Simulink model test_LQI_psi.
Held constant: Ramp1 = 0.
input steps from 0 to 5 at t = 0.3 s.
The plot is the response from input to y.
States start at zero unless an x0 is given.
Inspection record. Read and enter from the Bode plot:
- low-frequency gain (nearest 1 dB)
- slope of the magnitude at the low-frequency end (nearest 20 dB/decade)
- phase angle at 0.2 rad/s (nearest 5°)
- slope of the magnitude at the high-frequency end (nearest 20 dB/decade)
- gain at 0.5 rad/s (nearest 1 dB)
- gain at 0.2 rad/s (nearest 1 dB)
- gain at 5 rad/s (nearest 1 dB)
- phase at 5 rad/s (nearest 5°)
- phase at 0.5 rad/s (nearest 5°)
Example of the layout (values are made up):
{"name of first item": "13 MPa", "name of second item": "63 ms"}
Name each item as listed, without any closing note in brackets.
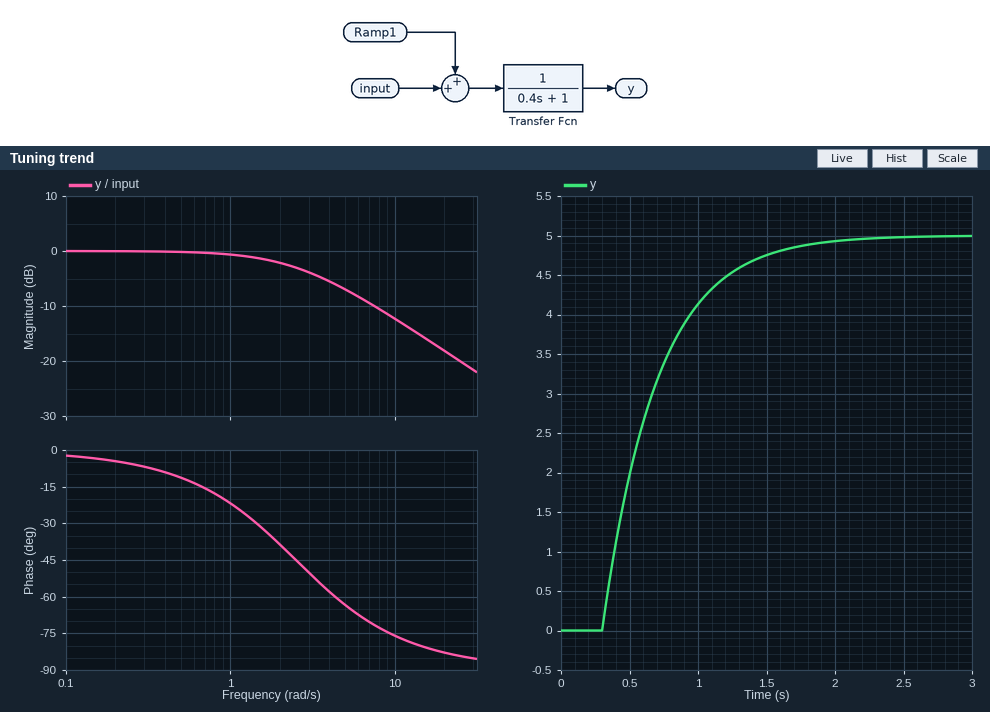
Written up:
{"low-frequency gain": "0 dB", "slope of the magnitude at the low-frequency end": "0 dB/decade", "phase angle at 0.2 rad/s": "-5°", "slope of the magnitude at the high-frequency end": "-20 dB/decade", "gain at 0.5 rad/s": "0 dB", "gain at 0.2 rad/s": "0 dB", "gain at 5 rad/s": "-7 dB", "phase at 5 rad/s": "-65°", "phase at 0.5 rad/s": "-10°"}
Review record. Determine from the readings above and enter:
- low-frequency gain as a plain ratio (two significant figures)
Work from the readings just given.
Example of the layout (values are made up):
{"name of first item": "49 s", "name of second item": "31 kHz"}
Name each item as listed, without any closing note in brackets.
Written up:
{"low-frequency gain as a plain ratio": "1.0"}
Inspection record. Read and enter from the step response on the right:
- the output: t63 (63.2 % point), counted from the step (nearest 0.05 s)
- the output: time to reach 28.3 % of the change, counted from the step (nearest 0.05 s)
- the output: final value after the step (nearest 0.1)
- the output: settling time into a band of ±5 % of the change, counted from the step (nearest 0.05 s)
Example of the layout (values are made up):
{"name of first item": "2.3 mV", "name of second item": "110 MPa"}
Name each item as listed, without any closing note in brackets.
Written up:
{"the output: t63 (63.2 % point), counted from the step": "0.40 s", "the output: time to reach 28.3 % of the change, counted from the step": "0.15 s", "the output: final value after the step": "5.0", "the output: settling time into a band of ±5 % of the change, counted from the step": "1.20 s"}
